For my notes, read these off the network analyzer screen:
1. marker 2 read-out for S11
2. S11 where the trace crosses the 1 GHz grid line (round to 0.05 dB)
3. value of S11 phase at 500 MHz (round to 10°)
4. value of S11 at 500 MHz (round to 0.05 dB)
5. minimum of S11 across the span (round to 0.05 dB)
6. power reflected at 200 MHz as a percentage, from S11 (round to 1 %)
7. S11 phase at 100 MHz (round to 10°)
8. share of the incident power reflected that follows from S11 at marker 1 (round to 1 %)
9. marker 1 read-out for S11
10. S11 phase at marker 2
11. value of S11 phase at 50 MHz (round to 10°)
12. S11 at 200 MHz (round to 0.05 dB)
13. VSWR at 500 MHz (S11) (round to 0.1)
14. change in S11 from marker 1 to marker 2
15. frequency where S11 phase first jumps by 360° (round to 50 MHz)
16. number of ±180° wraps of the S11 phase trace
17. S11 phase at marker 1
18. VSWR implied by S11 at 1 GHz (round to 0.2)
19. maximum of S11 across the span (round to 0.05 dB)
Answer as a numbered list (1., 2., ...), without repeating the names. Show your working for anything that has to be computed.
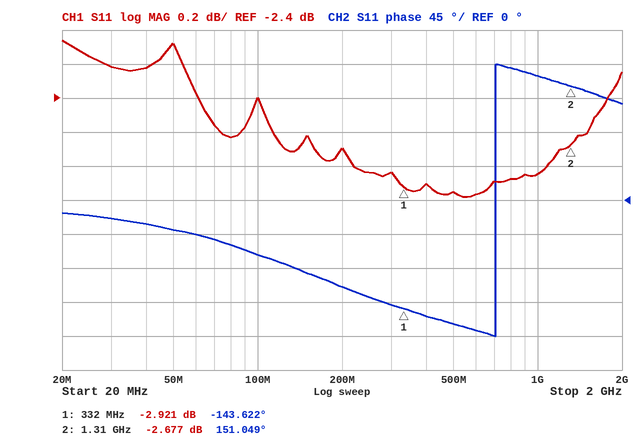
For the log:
1. -2.677 dB
2. -2.85 dB
3. -160°
4. -2.95 dB
5. -3.00 dB
6. 10^(-2.7/10) ≈ 54 %
7. -70°
8. 10^(-2.921/10) ≈ 51 %
9. -2.921 dB
10. 151.049°
11. -40°
12. -2.70 dB
13. |Γ| = 10^(-2.95/20) = 0.7120; VSWR = (1 + 0.7120)/(1 − 0.7120) ≈ 5.9
14. -2.677 − (-2.921) = 0.244 dB
15. 700 MHz
16. 1
17. -143.622°
18. |Γ| = 10^(-2.85/20) = 0.7203; VSWR = (1 + 0.7203)/(1 − 0.7203) ≈ 6.2
19. -2.05 dB
